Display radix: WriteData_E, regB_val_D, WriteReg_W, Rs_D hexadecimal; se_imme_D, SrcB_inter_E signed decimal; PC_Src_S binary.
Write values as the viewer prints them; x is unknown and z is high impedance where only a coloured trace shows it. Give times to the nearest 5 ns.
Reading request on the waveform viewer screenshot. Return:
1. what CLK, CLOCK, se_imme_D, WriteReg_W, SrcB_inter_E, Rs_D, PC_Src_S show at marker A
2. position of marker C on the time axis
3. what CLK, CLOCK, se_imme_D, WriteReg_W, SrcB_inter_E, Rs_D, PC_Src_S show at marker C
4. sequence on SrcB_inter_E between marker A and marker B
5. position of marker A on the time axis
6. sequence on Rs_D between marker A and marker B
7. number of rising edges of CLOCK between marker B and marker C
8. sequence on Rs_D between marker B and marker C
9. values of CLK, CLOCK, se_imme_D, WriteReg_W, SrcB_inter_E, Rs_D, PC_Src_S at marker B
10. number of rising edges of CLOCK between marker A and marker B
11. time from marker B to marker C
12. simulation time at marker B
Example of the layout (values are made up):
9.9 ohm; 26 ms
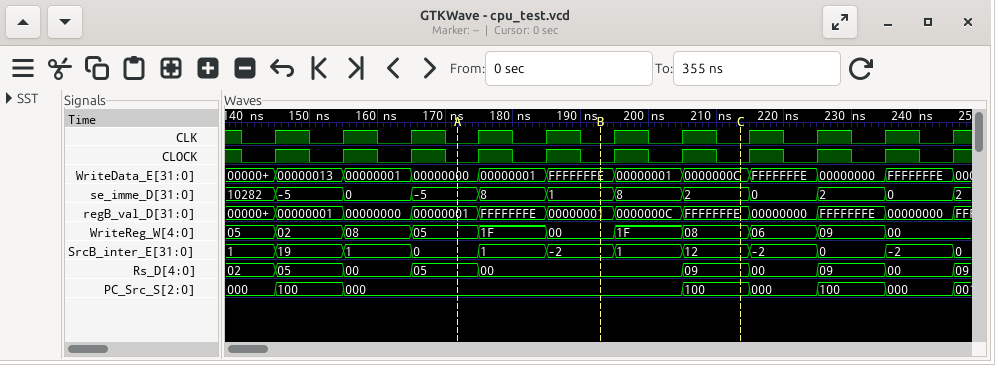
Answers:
CLK=0, CLOCK=0, se_imme_D=-5, WriteReg_W=05, SrcB_inter_E=0, Rs_D=05, PC_Src_S=000; 215 ns; CLK=0, CLOCK=0, se_imme_D=2, WriteReg_W=08, SrcB_inter_E=12, Rs_D=09, PC_Src_S=100; 0, 1, -2; 170 ns; 05, 00; 2; 00, 09; CLK=0, CLOCK=0, se_imme_D=1, WriteReg_W=00, SrcB_inter_E=-2, Rs_D=00, PC_Src_S=000; 2; 20 ns; 195 ns
